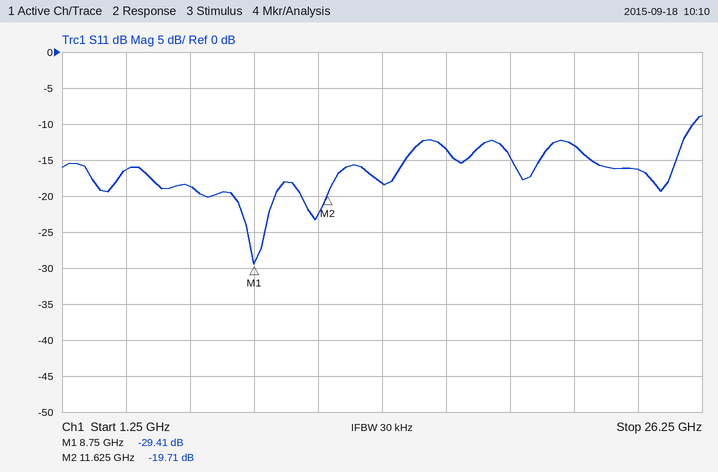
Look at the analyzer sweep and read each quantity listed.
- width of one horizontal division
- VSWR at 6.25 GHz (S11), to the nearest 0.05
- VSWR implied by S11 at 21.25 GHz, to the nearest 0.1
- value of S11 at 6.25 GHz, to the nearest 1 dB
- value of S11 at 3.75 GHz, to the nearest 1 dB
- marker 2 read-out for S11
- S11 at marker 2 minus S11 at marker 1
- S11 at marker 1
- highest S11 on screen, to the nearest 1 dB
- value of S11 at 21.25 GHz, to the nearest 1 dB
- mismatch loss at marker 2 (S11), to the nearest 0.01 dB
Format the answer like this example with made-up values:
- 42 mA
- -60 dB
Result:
- 2.5 GHz
- 1.25
- 1.6
- -19 dB
- -16 dB
- -19.71 dB
- 9.70 dB
- -29.41 dB
- -9 dB
- -13 dB
- 0.05 dB
